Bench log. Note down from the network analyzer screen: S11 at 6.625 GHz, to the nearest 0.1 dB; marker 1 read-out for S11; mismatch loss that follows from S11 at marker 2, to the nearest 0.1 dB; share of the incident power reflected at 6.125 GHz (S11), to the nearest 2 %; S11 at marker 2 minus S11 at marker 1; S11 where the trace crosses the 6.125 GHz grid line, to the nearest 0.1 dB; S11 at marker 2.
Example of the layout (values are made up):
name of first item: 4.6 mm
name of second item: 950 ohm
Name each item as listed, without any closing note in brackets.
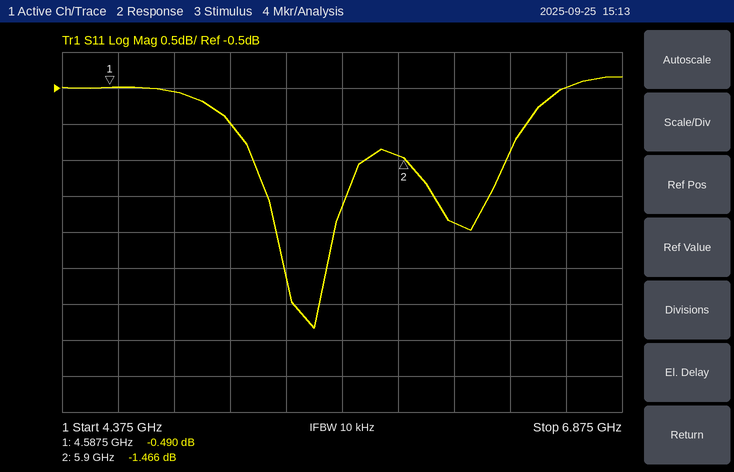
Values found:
S11 at 6.625 GHz, to the nearest 0.1 dB: -0.5 dB
marker 1 read-out for S11: -0.490 dB
mismatch loss that follows from S11 at marker 2, to the nearest 0.1 dB: 5.4 dB
share of the incident power reflected at 6.125 GHz (S11), to the nearest 2 %: 58 %
S11 at marker 2 minus S11 at marker 1: -0.976 dB
S11 where the trace crosses the 6.125 GHz grid line, to the nearest 0.1 dB: -2.4 dB
S11 at marker 2: -1.466 dB
